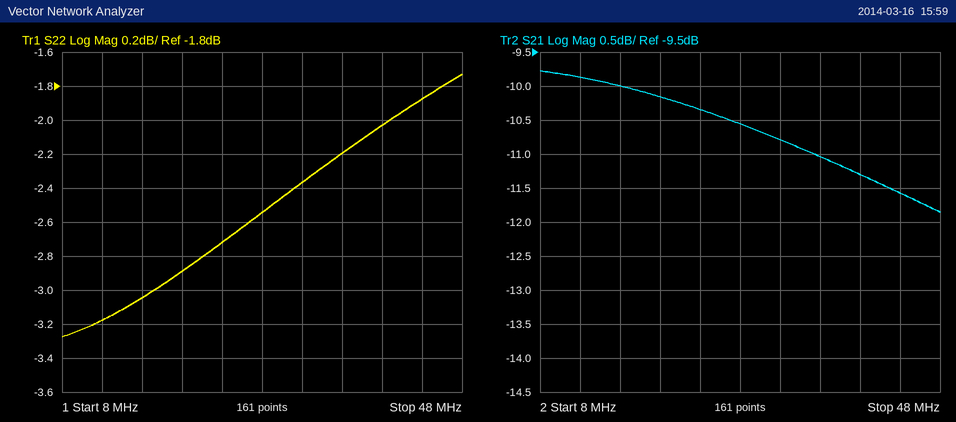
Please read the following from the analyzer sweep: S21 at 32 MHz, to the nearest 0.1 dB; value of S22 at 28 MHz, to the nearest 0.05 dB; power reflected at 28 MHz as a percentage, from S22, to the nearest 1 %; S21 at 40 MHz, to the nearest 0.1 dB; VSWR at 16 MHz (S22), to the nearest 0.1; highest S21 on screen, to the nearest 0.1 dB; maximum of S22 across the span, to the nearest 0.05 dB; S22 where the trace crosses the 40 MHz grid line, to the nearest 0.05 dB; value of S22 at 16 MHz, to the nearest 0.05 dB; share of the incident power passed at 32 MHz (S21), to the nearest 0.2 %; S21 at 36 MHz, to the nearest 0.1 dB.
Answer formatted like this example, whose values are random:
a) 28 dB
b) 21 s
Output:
a) -10.8 dB
b) -2.55 dB
c) 56 %
d) -11.3 dB
e) 5.8
f) -9.8 dB
g) -1.75 dB
h) -2.05 dB
i) -3.05 dB
j) 8.4 %
k) -11.0 dB
